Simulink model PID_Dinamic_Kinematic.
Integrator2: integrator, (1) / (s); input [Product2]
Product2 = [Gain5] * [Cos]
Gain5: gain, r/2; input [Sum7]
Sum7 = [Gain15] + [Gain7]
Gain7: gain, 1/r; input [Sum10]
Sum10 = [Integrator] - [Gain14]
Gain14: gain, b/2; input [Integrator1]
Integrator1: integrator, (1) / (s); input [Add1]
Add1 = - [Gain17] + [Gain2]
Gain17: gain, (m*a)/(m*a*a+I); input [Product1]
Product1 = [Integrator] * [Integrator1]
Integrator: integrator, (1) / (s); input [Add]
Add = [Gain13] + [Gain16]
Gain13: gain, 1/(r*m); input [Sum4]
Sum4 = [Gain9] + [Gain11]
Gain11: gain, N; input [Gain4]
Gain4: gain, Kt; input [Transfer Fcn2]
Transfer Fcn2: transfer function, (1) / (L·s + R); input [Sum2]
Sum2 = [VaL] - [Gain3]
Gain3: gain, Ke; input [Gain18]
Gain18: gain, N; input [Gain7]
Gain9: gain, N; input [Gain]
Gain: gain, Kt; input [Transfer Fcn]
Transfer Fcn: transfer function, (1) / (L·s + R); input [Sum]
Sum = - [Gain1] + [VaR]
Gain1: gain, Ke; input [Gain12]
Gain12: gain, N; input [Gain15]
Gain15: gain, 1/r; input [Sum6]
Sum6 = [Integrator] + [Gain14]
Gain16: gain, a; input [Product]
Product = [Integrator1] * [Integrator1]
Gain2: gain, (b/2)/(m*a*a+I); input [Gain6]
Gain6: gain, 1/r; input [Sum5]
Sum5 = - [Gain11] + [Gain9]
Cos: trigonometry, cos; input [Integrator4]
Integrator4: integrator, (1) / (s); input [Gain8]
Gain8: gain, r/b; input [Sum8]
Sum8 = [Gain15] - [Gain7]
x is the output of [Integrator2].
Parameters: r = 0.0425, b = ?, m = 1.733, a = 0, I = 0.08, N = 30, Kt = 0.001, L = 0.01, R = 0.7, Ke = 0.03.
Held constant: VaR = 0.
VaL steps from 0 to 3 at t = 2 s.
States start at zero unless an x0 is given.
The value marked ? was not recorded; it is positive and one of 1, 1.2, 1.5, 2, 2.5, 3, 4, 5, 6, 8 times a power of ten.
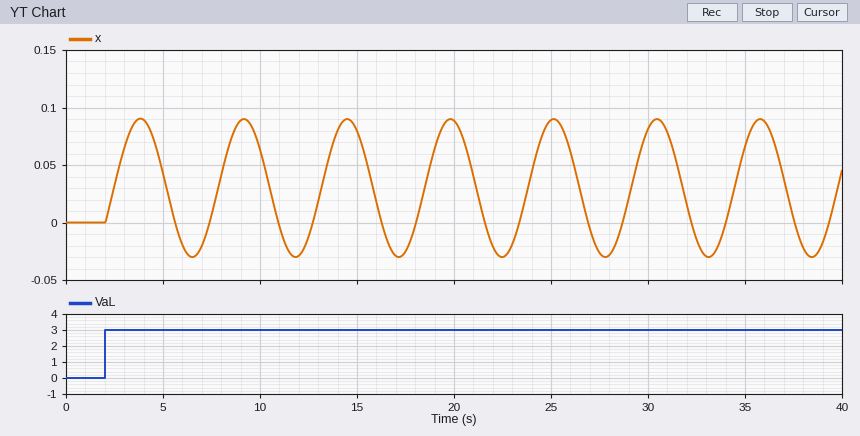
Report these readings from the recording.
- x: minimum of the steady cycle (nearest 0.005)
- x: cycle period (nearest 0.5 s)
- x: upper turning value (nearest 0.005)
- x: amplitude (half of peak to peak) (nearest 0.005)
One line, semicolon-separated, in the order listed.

-0.030; 5.5 s; 0.090; 0.060
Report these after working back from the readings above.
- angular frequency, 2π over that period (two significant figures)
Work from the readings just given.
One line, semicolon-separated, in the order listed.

1.1 rad/s
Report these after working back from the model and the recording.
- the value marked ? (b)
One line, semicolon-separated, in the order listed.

0.12
